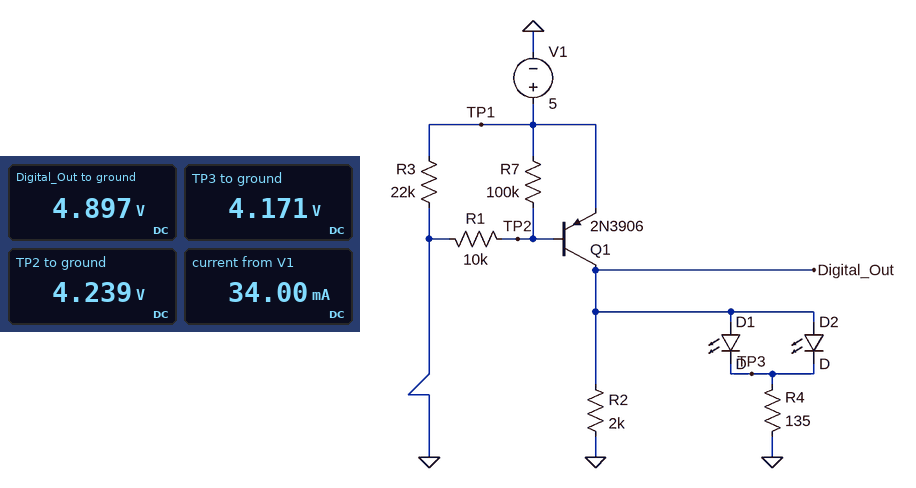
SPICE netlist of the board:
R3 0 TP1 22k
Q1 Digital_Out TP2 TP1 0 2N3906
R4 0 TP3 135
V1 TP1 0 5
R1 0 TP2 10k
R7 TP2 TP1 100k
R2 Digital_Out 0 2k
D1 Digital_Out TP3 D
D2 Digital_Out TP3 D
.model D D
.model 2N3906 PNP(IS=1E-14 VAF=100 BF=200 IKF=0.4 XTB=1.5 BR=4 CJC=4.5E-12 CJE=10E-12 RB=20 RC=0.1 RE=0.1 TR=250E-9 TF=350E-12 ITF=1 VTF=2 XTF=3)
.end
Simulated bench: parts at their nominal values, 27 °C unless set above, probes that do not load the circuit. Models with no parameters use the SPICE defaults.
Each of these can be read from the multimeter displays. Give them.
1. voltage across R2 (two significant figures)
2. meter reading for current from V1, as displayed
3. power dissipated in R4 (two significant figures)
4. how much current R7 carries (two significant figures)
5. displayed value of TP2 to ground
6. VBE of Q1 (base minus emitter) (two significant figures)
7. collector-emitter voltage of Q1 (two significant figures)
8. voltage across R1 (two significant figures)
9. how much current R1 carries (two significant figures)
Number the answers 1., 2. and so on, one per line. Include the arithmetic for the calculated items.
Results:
1. 4.897 V = 4.9 V
2. 34.00 mA
3. (4.171 V)^2 / 135 Ω = 130 mW
4. (5 V - 4.239 V) / 100 kΩ = 7.6 µA
5. 4.239 V
6. 4.239 V - 5 V = -760 mV
7. 4.897 V - 5 V = -100 mV
8. 4.239 V = 4.2 V
9. (4.239 V) / 10 kΩ = 420 µA
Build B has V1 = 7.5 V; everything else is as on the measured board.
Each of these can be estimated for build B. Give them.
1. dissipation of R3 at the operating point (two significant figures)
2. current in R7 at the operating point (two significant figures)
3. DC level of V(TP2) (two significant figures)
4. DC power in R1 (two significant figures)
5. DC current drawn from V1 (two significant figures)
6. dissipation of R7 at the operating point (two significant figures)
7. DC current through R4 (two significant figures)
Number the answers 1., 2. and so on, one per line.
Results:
1. 2.6 mW
2. 7.8 µA
3. 6.7 V
4. 4.5 mW
5. 54 mA
6. 6.1 µW
7. 49 mA
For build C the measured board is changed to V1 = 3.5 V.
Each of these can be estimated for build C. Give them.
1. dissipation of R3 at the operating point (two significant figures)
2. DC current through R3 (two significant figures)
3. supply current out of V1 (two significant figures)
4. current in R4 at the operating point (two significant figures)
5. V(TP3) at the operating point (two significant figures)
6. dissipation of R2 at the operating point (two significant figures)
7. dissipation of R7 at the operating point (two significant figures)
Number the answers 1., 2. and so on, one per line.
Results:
1. 560 µW
2. 160 µA
3. 22 mA
4. 20 mA
5. 2.7 V
6. 5.8 mW
7. 5.5 µW
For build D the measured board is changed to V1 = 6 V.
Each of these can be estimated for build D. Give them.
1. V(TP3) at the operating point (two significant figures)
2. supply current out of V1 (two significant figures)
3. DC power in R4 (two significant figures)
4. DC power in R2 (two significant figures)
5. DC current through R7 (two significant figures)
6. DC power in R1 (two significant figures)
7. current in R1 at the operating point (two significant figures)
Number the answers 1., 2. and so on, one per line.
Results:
1. 5.2 V
2. 42 mA
3. 200 mW
4. 17 mW
5. 7.7 µA
6. 2.7 mW
7. 520 µA
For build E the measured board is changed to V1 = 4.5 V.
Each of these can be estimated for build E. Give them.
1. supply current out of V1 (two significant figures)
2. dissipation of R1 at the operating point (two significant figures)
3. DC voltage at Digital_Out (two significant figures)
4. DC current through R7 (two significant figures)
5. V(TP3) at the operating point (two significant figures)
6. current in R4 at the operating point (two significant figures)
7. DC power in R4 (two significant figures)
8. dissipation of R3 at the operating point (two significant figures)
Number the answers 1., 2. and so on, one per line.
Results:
1. 30 mA
2. 1.4 mW
3. 4.4 V
4. 7.6 µA
5. 3.7 V
6. 27 mA
7. 100 mW
8. 920 µW
